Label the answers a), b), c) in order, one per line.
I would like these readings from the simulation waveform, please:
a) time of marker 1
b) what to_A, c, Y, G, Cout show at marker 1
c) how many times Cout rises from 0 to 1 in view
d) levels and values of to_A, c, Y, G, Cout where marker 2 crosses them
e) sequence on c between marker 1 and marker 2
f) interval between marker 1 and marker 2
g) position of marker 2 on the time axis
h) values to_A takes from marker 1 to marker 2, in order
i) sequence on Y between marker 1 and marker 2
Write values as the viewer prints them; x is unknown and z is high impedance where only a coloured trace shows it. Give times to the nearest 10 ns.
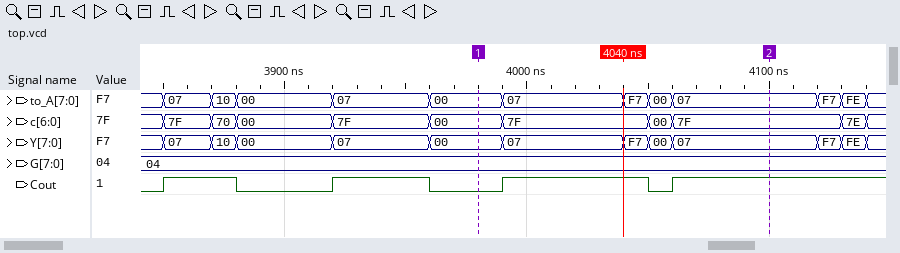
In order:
a) 3980 ns
b) to_A=00, c=00, Y=00, G=04, Cout=0
c) 4
d) to_A=07, c=7F, Y=07, G=04, Cout=1
e) 00, 7F, 00, 7F
f) 120 ns
g) 4100 ns
h) 00, 07, F7, 00, 07
i) 00, 07, F7, 00, 07
